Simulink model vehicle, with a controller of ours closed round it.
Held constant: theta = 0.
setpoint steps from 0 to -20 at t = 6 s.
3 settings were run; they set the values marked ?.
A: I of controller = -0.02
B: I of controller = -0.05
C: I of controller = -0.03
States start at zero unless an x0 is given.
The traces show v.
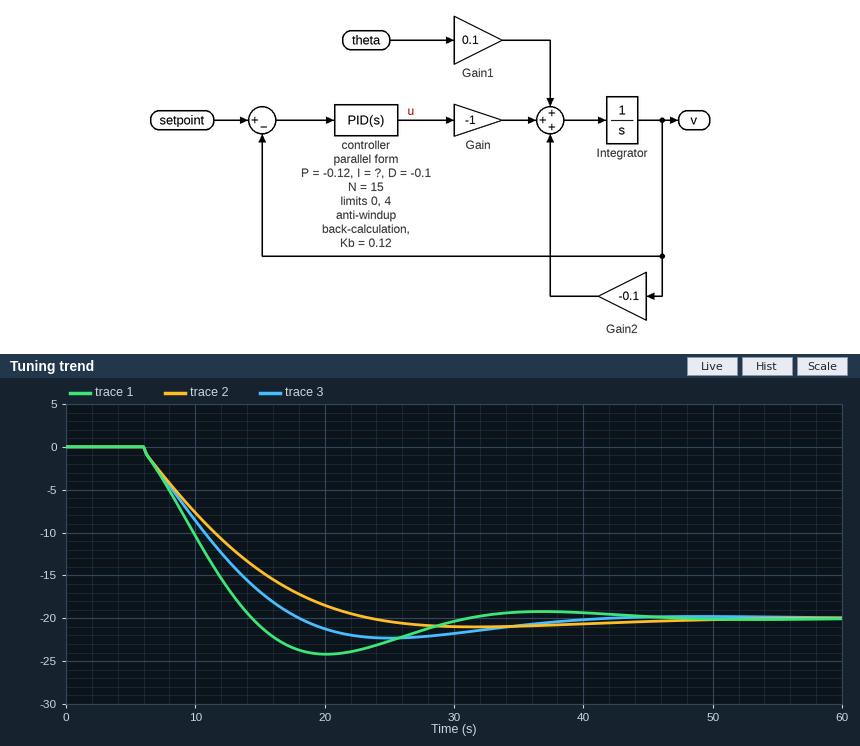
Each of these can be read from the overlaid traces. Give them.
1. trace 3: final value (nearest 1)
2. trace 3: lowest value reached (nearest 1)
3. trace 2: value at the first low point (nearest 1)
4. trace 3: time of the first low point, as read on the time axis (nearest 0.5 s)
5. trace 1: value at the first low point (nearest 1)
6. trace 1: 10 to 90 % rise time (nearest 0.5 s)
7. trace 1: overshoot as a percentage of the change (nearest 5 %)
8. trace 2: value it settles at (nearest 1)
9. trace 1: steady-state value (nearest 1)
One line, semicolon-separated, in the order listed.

-20; -22; -21; 25.0 s; -24; 6.5 s; 20 %; -20; -20
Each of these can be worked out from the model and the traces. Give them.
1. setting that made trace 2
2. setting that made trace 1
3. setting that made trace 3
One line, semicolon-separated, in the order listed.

A; B; C
